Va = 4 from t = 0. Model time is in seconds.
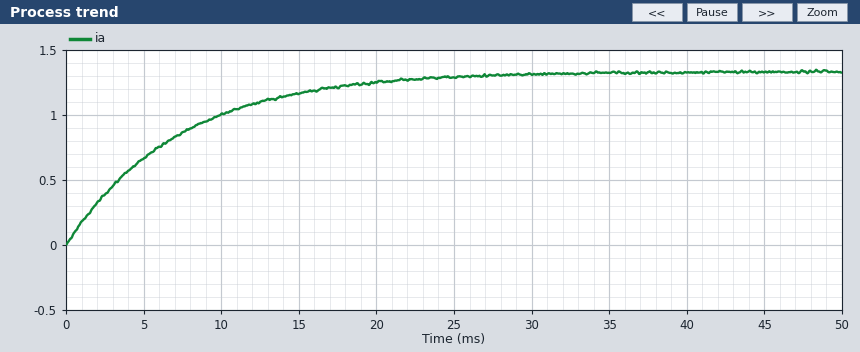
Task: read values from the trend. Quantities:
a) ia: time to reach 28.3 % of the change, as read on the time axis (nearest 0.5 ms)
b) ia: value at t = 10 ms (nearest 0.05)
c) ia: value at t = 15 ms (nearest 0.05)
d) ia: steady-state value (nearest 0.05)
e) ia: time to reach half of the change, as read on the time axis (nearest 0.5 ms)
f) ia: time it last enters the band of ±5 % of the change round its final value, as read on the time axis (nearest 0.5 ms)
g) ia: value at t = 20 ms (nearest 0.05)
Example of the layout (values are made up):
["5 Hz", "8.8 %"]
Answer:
["2.5 ms", "1.00", "1.15", "1.35", "5.0 ms", "21.5 ms", "1.25"]
